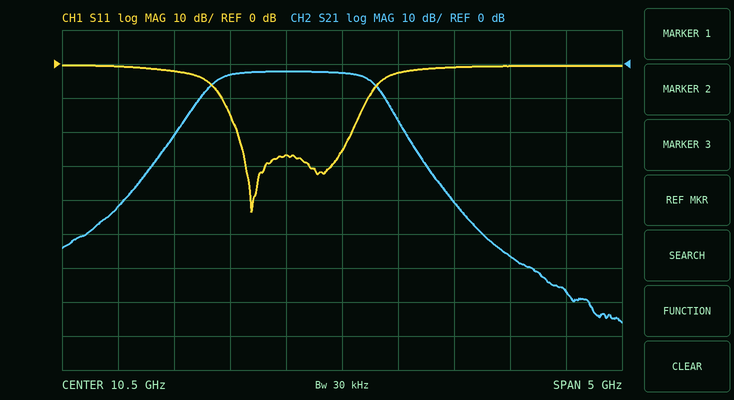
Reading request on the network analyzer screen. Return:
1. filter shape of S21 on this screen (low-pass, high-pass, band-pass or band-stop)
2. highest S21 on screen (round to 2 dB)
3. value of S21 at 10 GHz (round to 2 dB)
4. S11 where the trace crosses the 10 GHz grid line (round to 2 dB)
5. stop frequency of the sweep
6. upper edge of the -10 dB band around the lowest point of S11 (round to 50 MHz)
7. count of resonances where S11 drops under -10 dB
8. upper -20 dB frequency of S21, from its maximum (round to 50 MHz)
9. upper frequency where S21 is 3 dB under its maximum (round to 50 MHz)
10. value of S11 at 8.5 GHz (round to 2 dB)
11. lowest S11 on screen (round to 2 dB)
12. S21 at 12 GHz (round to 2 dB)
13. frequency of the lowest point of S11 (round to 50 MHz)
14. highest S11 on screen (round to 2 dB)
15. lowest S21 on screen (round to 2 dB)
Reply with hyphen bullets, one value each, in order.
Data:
- band-pass
- -2 dB
- -2 dB
- -26 dB
- 13 GHz
- 10.75 GHz
- 2
- 11.10 GHz
- 10.75 GHz
- 0 dB
- -44 dB
- -56 dB
- 9.70 GHz
- 0 dB
- -76 dB
